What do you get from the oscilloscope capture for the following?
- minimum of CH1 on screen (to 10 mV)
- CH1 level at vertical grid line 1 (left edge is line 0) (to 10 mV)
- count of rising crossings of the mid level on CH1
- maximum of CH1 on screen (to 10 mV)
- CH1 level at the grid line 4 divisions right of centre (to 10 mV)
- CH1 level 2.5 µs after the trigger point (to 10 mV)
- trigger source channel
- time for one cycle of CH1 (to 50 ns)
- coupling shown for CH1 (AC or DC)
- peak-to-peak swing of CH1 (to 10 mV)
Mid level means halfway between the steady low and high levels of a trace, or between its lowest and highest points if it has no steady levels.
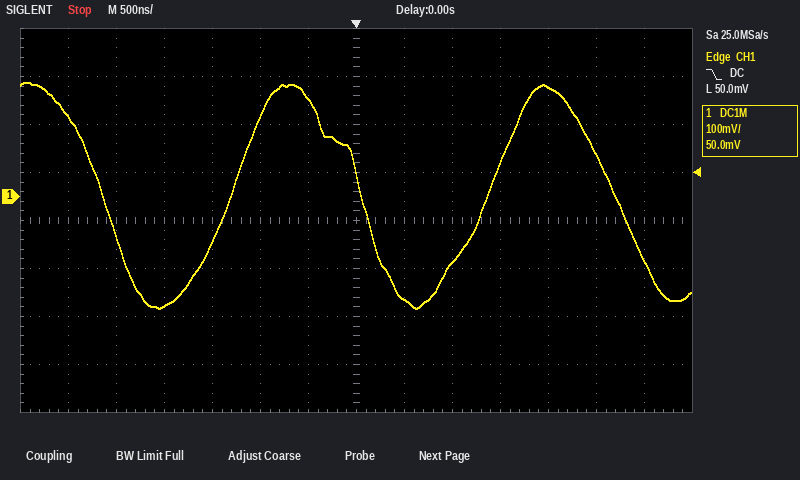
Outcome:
-230 mV
170 mV
2
240 mV
230 mV
90 mV
CH1
2.65 µs
DC
470 mV
